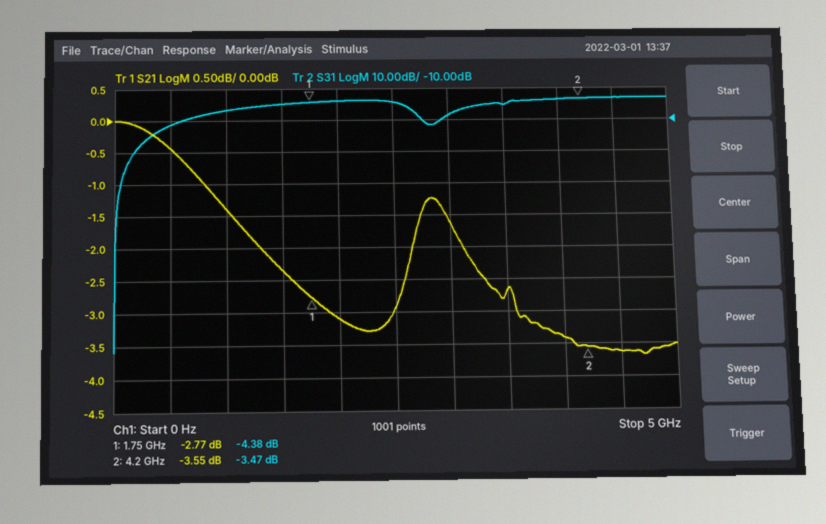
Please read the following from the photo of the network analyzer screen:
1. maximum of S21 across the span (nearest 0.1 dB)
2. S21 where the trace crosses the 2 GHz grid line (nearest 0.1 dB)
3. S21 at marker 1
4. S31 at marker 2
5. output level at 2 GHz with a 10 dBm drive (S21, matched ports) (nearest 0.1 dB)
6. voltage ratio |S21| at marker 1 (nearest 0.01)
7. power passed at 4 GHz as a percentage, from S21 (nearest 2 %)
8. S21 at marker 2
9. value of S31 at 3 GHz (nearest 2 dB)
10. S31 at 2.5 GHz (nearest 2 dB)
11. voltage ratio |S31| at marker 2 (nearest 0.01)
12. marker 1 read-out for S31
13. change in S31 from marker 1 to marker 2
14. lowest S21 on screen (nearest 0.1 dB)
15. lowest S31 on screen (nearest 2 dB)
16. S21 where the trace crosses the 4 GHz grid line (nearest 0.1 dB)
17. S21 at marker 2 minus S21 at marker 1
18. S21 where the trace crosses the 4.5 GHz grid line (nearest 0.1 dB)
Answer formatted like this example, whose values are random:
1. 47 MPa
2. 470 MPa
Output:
1. 0.0 dB
2. -3.1 dB
3. -2.77 dB
4. -3.47 dB
5. 6.9 dBm
6. 0.73
7. 46 %
8. -3.55 dB
9. -8 dB
10. -4 dB
11. 0.67
12. -4.38 dB
13. 0.91 dB
14. -3.7 dB
15. -82 dB
16. -3.4 dB
17. -0.78 dB
18. -3.6 dB
